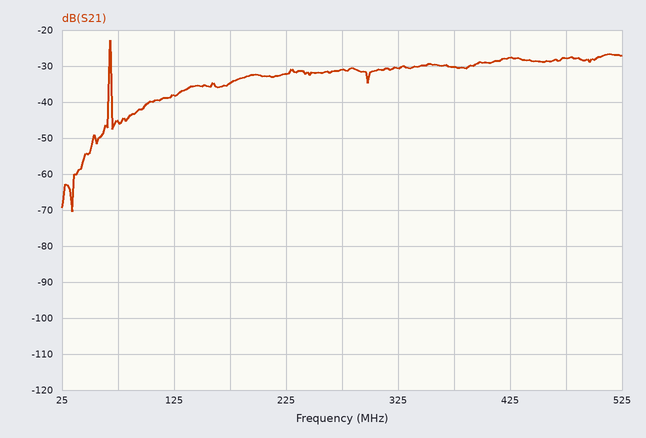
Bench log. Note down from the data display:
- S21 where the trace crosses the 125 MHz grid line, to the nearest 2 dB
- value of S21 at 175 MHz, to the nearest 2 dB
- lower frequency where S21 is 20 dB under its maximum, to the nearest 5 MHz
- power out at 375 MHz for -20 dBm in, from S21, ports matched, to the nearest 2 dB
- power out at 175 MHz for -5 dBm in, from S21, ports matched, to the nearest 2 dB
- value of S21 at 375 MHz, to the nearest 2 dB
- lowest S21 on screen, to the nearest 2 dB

-38 dB
-34 dB
65 MHz
-50 dBm
-40 dBm
-30 dB
-70 dB
